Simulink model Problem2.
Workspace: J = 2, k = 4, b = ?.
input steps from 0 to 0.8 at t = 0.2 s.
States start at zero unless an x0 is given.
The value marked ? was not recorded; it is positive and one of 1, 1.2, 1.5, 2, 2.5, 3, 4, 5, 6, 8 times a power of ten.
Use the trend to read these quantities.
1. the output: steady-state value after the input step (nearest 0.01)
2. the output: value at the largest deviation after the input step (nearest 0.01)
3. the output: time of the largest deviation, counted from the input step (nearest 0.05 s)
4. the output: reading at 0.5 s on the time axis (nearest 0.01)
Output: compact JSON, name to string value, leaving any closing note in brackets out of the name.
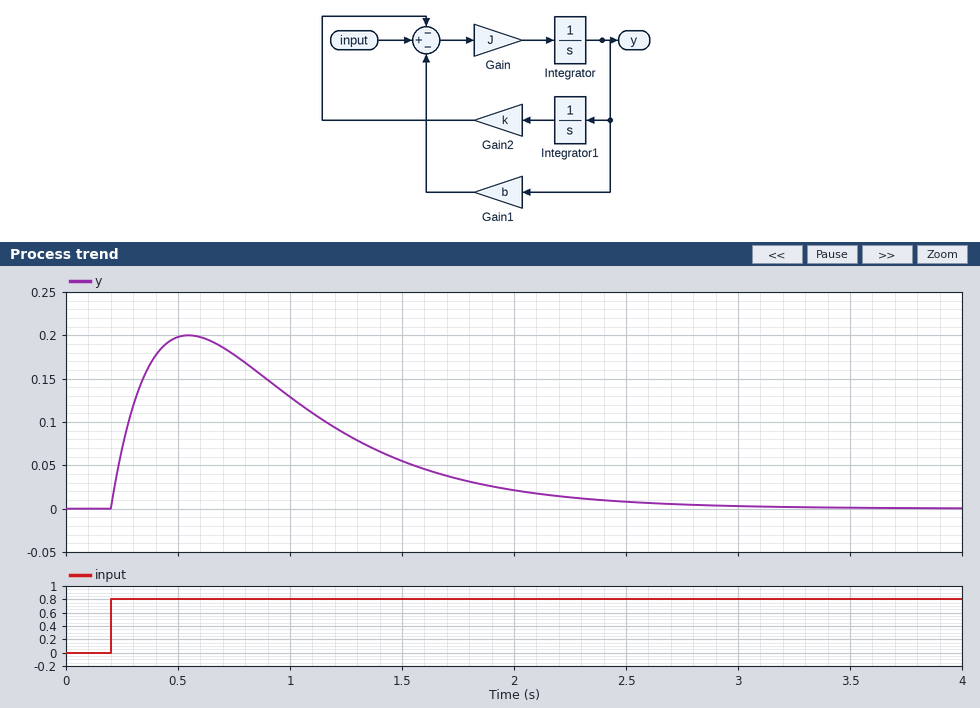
{"the output: steady-state value after the input step": "0.00", "the output: value at the largest deviation after the input step": "0.20", "the output: time of the largest deviation, counted from the input step": "0.35 s", "the output: reading at 0.5 s on the time axis": "0.20"}
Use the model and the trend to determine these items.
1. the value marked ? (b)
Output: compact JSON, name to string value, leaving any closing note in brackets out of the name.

{"the value marked ?": "3"}
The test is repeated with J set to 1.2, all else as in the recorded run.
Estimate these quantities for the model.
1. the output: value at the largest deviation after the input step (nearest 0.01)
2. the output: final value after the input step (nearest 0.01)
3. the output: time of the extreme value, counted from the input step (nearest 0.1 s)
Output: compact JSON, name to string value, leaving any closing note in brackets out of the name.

{"the output: value at the largest deviation after the input step": "0.18", "the output: final value after the input step": "0.00", "the output: time of the extreme value, counted from the input step": "0.5 s"}
